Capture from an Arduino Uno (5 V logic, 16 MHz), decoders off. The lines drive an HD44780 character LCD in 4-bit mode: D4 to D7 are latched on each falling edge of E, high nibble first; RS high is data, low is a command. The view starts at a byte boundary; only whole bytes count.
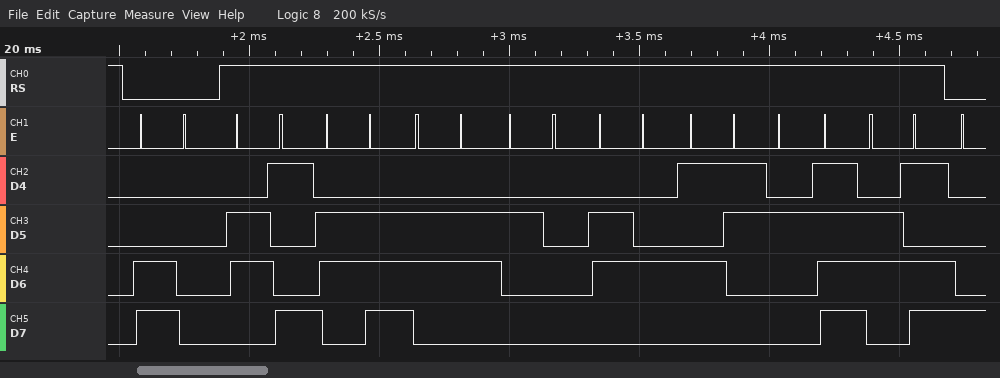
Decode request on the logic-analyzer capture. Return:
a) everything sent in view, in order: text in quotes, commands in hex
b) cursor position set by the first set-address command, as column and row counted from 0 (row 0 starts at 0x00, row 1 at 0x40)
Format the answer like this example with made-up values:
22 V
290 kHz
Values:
0xC0 "inf dS/m"
column 0, row 1
